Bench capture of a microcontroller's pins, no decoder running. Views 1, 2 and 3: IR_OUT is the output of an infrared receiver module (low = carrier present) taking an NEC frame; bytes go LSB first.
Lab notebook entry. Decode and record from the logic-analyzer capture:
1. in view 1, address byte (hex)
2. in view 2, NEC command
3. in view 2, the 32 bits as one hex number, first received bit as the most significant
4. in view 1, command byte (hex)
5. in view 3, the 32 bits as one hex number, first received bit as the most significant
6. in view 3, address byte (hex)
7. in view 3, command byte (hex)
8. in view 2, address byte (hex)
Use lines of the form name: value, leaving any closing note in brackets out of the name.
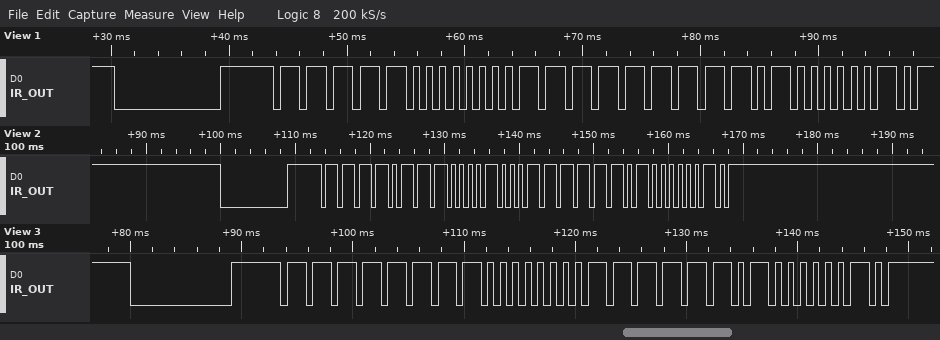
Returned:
in view 1, address byte: 0x1F
in view 2, NEC command: 0xBF
in view 2, the 32 bits as one hex number, first received bit as the most significant: 0xF708FD02
in view 1, command byte: 0xBF
in view 3, the 32 bits as one hex number, first received bit as the most significant: 0xFF00FD02
in view 3, address byte: 0xFF
in view 3, command byte: 0xBF
in view 2, address byte: 0xEF
